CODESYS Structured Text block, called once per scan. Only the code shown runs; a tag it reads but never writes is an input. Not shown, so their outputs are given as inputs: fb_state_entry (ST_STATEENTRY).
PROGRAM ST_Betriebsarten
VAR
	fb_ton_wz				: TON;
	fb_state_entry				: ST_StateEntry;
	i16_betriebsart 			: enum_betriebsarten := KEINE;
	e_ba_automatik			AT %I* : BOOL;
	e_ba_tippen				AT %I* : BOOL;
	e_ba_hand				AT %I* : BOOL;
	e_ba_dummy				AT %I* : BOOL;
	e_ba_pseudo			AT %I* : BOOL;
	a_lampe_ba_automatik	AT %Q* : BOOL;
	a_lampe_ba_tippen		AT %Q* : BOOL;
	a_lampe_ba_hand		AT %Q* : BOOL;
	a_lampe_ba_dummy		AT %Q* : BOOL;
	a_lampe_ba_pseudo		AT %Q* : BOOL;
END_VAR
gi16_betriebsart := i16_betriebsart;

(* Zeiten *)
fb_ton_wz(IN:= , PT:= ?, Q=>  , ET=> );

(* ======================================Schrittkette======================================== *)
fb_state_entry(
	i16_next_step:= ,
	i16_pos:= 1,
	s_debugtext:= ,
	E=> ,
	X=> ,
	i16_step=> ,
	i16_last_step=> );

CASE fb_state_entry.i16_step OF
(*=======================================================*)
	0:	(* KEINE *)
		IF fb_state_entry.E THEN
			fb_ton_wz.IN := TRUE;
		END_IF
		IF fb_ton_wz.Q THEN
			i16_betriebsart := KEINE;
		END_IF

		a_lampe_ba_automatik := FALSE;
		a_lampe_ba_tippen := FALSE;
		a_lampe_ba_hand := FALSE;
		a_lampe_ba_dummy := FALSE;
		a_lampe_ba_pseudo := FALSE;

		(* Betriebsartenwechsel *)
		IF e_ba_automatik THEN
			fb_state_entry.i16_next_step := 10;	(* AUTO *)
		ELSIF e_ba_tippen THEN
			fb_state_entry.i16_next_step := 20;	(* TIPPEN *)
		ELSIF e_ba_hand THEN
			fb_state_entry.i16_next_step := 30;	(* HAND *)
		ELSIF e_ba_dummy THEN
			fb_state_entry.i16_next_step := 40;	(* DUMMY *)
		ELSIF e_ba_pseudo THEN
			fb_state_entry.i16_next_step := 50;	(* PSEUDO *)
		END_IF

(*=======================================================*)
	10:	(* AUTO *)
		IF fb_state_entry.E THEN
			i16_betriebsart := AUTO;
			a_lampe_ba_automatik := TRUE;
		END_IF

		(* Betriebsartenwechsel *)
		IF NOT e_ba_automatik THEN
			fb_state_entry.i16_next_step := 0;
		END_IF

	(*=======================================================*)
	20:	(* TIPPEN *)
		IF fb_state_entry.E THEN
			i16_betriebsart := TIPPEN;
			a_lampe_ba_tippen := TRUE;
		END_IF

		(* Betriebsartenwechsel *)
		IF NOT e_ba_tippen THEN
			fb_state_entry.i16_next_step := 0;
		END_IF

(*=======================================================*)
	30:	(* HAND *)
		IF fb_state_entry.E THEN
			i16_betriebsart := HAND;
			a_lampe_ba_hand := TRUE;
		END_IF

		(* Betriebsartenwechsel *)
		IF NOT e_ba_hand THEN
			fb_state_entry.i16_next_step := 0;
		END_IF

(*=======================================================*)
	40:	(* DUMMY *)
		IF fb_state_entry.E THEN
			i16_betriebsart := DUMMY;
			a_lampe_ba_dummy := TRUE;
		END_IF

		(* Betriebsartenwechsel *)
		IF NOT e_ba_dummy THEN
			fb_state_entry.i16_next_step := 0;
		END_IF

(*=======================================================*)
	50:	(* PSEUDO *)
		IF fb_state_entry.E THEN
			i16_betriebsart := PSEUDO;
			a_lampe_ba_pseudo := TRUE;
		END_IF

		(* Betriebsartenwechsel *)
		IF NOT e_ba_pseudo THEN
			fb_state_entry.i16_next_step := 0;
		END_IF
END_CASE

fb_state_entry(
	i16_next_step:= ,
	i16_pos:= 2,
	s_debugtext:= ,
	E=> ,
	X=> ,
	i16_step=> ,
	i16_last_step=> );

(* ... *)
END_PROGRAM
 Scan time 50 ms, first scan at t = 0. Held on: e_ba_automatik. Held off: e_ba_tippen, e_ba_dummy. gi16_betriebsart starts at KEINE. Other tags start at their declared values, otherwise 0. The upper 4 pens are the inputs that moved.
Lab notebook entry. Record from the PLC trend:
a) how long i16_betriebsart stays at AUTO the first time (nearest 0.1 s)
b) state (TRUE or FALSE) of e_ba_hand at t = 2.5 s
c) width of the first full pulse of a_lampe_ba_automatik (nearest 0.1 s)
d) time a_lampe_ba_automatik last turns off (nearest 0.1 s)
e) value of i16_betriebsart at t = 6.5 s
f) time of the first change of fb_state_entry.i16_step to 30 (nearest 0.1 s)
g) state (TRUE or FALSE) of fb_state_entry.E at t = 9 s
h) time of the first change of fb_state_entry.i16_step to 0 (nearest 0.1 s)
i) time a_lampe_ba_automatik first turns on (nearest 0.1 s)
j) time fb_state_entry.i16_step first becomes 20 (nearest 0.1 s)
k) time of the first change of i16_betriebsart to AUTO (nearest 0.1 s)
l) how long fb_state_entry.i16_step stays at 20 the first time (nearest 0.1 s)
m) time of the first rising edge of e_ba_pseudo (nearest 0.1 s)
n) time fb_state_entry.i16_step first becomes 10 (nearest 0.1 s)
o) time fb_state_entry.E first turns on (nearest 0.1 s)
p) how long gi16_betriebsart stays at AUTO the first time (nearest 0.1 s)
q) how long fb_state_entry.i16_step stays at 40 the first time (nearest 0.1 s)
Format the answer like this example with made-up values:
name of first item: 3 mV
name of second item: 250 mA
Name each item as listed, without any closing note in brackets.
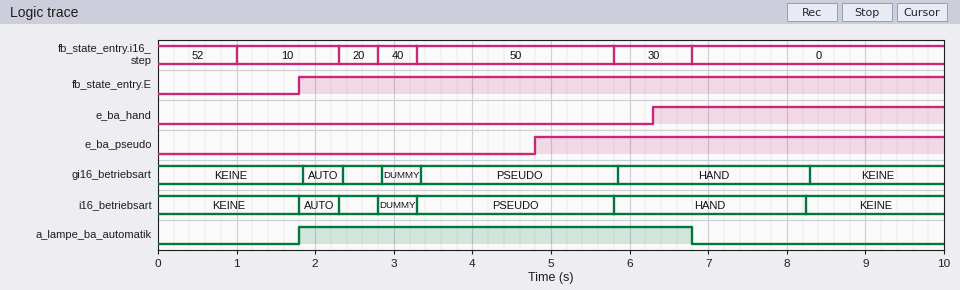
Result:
how long i16_betriebsart stays at AUTO the first time: 0.5 s
state (TRUE or FALSE) of e_ba_hand at t = 2.5 s: FALSE
width of the first full pulse of a_lampe_ba_automatik: 5.0 s
time a_lampe_ba_automatik last turns off: 6.8 s
value of i16_betriebsart at t = 6.5 s: HAND
time of the first change of fb_state_entry.i16_step to 30: 5.8 s
state (TRUE or FALSE) of fb_state_entry.E at t = 9 s: TRUE
time of the first change of fb_state_entry.i16_step to 0: 6.8 s
time a_lampe_ba_automatik first turns on: 1.8 s
time fb_state_entry.i16_step first becomes 20: 2.3 s
time of the first change of i16_betriebsart to AUTO: 1.8 s
how long fb_state_entry.i16_step stays at 20 the first time: 0.5 s
time of the first rising edge of e_ba_pseudo: 4.8 s
time fb_state_entry.i16_step first becomes 10: 1.0 s
time fb_state_entry.E first turns on: 1.8 s
how long gi16_betriebsart stays at AUTO the first time: 0.5 s
how long fb_state_entry.i16_step stays at 40 the first time: 0.5 s
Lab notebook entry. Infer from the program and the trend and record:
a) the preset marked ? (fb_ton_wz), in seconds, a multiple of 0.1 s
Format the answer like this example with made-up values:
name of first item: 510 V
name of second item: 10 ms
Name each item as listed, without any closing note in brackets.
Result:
the preset marked ? (fb_ton_wz), in seconds, a multiple of 0.1 s: 1.4 s
